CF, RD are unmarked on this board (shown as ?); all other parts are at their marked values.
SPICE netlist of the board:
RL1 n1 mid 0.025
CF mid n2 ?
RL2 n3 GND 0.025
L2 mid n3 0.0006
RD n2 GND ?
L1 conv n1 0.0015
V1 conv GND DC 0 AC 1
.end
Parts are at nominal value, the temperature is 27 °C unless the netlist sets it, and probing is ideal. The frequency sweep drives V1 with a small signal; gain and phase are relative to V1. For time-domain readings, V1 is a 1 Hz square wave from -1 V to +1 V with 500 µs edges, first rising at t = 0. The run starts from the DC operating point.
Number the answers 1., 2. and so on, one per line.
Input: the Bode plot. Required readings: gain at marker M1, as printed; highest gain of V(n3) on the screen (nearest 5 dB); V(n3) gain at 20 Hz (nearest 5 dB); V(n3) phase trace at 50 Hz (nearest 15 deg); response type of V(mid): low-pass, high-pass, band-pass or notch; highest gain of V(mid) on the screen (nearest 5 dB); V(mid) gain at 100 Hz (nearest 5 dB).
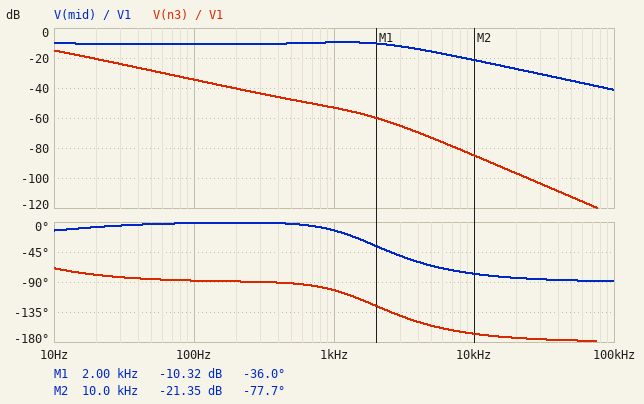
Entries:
1. -10.32 dB
2. -15 dB
3. -20 dB
4. -90 deg
5. low-pass
6. -10 dB
7. -10 dB
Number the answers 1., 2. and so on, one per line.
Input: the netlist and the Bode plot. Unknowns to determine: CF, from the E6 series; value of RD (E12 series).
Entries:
1. 22 µF
2. 8.2 Ω
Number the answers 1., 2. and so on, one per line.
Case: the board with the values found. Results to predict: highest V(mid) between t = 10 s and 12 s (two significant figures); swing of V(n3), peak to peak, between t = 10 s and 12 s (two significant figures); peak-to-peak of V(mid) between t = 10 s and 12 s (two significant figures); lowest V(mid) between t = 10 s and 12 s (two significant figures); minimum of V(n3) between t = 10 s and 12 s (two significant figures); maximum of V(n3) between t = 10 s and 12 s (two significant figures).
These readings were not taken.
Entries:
1. 500 mV
2. 1.0 V
3. 1.0 V
4. -500 mV
5. -500 mV
6. 500 mV
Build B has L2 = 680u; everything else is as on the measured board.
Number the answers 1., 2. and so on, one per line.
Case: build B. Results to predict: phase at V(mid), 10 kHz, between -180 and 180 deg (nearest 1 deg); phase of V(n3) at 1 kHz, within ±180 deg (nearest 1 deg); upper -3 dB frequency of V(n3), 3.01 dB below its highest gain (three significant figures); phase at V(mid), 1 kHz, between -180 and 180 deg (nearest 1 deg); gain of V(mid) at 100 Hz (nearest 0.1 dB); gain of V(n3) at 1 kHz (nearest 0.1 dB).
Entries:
1. -79 deg
2. -104 deg
3. 3.65 Hz
4. -14 deg
5. -10.1 dB
6. -53.3 dB
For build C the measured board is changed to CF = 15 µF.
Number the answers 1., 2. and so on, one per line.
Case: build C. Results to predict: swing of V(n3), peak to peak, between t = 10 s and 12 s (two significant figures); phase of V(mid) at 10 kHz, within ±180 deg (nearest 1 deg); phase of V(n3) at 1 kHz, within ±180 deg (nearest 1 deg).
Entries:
1. 1.0 V
2. -80 deg
3. -98 deg
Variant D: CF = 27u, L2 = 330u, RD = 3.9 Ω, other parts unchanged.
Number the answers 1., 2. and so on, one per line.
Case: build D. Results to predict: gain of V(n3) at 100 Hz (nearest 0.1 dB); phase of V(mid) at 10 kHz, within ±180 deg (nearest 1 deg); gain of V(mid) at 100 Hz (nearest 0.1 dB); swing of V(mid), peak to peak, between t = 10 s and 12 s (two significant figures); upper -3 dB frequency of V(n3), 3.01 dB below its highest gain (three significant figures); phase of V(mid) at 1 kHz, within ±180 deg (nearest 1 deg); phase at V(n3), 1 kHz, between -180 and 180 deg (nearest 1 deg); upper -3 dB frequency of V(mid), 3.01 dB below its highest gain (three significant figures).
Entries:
1. -33.2 dB
2. -85 deg
3. -14.8 dB
4. 1.0 V
5. 4.35 Hz
6. -10 deg
7. -99 deg
8. 5.06 Hz
